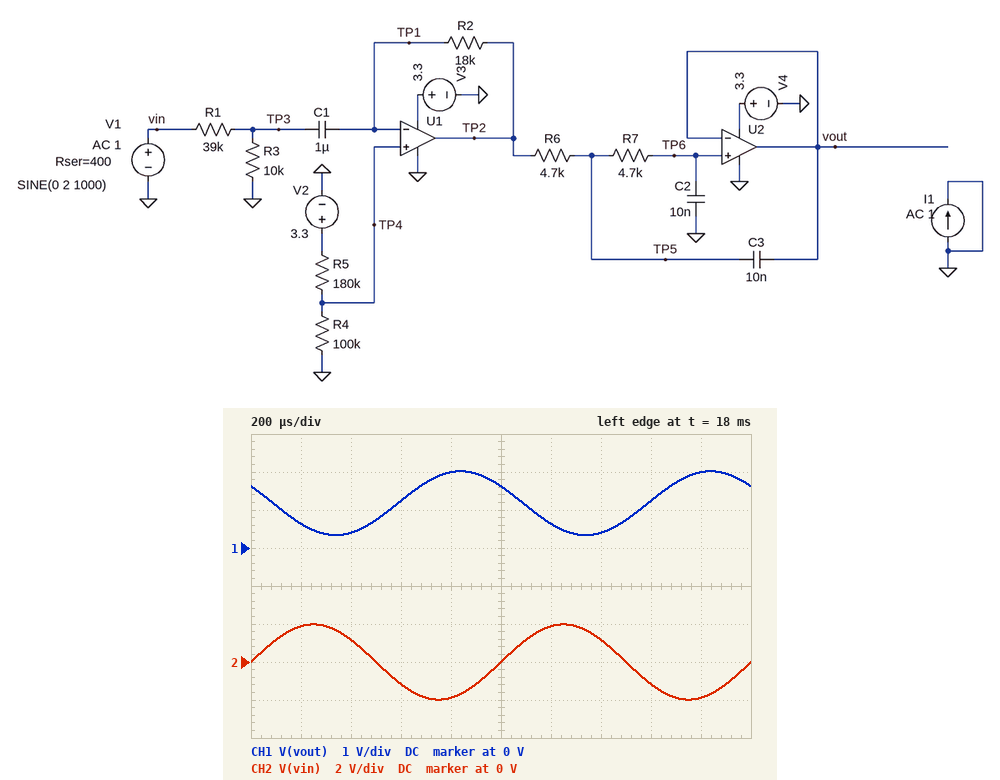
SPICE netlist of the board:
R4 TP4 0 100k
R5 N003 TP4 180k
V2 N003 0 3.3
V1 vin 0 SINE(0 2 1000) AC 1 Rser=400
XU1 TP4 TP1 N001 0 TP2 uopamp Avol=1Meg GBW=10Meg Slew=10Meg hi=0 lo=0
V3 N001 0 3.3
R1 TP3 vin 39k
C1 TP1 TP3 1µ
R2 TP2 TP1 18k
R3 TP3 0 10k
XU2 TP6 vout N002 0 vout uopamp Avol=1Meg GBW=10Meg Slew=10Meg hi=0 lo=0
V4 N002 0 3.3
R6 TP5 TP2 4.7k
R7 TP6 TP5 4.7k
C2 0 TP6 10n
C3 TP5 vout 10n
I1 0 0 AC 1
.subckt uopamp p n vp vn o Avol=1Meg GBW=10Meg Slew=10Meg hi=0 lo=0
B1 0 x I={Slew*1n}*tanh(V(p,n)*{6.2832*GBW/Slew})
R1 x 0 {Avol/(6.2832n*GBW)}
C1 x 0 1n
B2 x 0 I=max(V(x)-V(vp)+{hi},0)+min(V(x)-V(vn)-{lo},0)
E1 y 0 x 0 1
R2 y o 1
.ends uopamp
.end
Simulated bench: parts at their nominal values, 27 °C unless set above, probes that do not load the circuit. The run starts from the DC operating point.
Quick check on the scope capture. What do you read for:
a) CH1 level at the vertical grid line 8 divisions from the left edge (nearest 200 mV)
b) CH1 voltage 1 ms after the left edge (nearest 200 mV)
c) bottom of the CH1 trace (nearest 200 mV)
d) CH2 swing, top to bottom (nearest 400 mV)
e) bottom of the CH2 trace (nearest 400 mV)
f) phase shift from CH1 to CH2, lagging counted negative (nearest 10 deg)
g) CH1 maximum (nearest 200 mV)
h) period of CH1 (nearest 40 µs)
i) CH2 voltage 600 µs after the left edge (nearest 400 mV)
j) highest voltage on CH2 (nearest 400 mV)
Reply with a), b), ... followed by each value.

a) 1.2 V
b) 1.6 V
c) 400 mV
d) 4.0 V
e) -2.0 V
f) -150 deg
g) 2.0 V
h) 1.00 ms
i) -1.2 V
j) 2.0 V
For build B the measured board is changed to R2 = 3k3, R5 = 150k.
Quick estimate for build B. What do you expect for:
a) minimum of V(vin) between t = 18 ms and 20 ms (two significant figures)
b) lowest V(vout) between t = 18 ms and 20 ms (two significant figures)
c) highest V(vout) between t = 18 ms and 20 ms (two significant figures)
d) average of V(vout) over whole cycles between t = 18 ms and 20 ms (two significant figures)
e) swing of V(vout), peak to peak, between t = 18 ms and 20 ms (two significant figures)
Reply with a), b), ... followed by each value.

a) -2.0 V
b) 1.2 V
c) 1.5 V
d) 1.3 V
e) 310 mV
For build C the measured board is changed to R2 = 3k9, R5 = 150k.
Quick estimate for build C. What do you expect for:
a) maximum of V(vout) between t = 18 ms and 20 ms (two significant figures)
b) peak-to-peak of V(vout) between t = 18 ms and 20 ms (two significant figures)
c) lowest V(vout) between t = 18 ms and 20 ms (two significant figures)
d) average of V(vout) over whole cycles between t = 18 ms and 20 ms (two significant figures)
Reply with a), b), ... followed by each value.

a) 1.5 V
b) 360 mV
c) 1.1 V
d) 1.3 V
